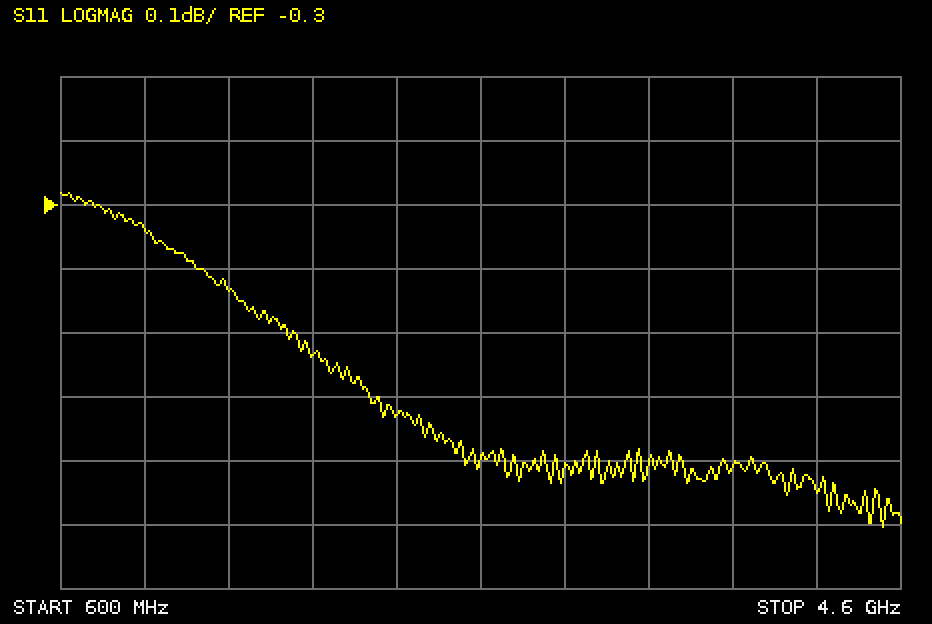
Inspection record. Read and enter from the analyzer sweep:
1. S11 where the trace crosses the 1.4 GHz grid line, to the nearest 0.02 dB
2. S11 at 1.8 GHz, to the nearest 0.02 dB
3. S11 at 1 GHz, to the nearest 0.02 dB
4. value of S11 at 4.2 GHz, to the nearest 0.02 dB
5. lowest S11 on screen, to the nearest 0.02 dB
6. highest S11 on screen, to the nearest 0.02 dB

-0.44 dB
-0.54 dB
-0.34 dB
-0.74 dB
-0.80 dB
-0.28 dB
